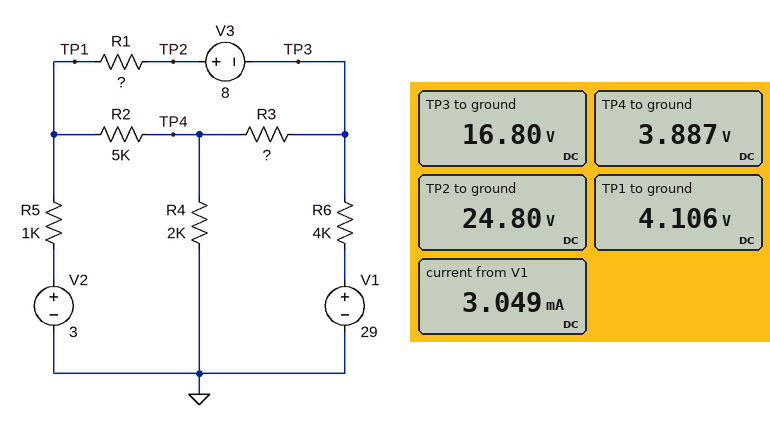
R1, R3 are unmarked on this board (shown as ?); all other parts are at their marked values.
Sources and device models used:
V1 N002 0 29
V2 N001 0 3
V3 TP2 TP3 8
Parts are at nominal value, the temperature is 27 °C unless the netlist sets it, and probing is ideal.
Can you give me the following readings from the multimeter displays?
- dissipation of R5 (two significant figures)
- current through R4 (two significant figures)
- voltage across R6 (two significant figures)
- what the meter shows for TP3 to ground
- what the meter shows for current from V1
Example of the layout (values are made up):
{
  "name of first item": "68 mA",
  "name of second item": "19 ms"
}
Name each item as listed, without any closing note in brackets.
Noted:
{
  "dissipation of R5": "1.2 mW",
  "current through R4": "1.9 mA",
  "voltage across R6": "12 V",
  "what the meter shows for TP3 to ground": "16.80 V",
  "what the meter shows for current from V1": "3.049 mA"
}
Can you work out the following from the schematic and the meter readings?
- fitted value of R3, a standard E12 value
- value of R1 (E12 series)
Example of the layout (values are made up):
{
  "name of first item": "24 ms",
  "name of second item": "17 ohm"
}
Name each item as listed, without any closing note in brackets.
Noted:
{
  "fitted value of R3, a standard E12 value": "6.8 kΩ",
  "value of R1": "18 kΩ"
}
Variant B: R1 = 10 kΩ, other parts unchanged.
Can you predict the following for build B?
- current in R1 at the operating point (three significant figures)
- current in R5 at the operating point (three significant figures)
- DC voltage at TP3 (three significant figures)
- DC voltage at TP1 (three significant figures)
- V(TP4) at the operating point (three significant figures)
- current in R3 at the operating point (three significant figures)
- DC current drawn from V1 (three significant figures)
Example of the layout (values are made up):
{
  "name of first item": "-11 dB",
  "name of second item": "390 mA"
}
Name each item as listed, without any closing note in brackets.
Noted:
{
  "current in R1 at the operating point": "1.84 mA",
  "current in R5 at the operating point": "1.65 mA",
  "DC voltage at TP3": "15.0 V",
  "DC voltage at TP1": "4.65 V",
  "V(TP4) at the operating point": "3.70 V",
  "current in R3 at the operating point": "1.66 mA",
  "DC current drawn from V1": "3.50 mA"
}
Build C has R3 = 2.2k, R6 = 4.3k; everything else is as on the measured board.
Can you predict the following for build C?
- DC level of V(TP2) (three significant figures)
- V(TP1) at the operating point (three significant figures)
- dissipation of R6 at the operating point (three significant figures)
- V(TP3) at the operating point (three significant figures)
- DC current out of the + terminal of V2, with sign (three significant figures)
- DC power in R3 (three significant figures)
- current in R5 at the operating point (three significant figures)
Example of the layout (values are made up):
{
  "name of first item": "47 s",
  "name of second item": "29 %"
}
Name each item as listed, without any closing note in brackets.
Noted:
{
  "DC level of V(TP2)": "20.2 V",
  "V(TP1) at the operating point": "4.16 V",
  "dissipation of R6 at the operating point": "65.9 mW",
  "V(TP3) at the operating point": "12.2 V",
  "DC current out of the + terminal of V2, with sign": "-1.16 mA",
  "DC power in R3": "20.1 mW",
  "current in R5 at the operating point": "1.16 mA"
}
